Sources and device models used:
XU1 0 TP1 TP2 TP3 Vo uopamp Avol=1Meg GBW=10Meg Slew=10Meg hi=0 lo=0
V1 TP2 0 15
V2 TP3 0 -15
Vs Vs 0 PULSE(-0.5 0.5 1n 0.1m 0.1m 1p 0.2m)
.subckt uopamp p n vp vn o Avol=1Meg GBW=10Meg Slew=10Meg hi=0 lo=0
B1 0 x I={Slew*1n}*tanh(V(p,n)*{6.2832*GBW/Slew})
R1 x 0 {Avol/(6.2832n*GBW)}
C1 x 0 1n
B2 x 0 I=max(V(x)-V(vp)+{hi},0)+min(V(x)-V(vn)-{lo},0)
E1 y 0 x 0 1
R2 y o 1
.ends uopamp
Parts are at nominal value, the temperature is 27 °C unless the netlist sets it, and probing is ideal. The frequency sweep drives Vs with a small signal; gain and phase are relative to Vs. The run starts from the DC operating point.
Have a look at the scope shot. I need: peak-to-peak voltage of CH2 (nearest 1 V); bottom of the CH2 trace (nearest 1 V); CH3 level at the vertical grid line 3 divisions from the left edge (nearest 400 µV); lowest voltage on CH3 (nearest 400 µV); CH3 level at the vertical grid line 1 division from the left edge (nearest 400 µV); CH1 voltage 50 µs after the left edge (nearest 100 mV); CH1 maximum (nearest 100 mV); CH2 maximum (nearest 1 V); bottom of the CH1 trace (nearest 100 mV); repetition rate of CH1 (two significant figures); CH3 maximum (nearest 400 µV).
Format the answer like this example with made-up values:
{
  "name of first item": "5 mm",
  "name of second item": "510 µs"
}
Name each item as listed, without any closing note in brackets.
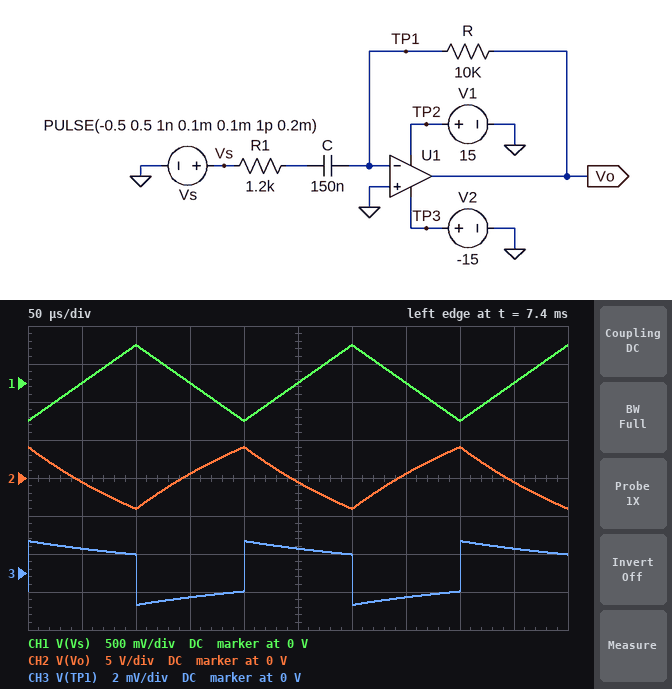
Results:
{
  "peak-to-peak voltage of CH2": "8 V",
  "bottom of the CH2 trace": "-4 V",
  "CH3 level at the vertical grid line 3 divisions from the left edge": "-1.2 mV",
  "lowest voltage on CH3": "-1.6 mV",
  "CH3 level at the vertical grid line 1 division from the left edge": "1.2 mV",
  "CH1 voltage 50 µs after the left edge": "0 V",
  "CH1 maximum": "500 mV",
  "CH2 maximum": "4 V",
  "bottom of the CH1 trace": "-500 mV",
  "repetition rate of CH1": "5.0 kHz",
  "CH3 maximum": "1.6 mV"
}
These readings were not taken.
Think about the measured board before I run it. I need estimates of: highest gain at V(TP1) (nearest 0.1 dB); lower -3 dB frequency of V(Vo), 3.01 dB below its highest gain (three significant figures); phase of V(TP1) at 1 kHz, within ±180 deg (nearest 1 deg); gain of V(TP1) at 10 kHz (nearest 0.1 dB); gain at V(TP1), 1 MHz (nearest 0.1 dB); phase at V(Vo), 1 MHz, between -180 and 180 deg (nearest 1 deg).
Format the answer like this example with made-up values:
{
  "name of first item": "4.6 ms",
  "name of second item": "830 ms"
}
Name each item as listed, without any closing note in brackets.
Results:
{
  "highest gain at V(TP1)": "-1.0 dB",
  "lower -3 dB frequency of V(Vo), 3.01 dB below its highest gain": "883 Hz",
  "phase of V(TP1) at 1 kHz, within ±180 deg": "131 deg",
  "gain of V(TP1) at 10 kHz": "-41.6 dB",
  "gain at V(TP1), 1 MHz": "-4.3 dB",
  "phase at V(Vo), 1 MHz, between -180 and 180 deg": "137 deg"
}
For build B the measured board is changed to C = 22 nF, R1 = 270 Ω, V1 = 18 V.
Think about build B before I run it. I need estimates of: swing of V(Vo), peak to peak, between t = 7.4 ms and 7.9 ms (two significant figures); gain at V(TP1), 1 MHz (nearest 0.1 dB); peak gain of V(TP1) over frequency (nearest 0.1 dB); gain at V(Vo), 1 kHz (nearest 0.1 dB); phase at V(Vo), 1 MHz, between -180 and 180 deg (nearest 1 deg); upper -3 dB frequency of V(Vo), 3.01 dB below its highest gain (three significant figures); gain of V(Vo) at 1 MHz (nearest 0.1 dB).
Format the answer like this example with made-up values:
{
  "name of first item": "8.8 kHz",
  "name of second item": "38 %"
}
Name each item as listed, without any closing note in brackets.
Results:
{
  "swing of V(Vo), peak to peak, between t = 7.4 ms and 7.9 ms": "4.4 V",
  "gain at V(TP1), 1 MHz": "-0.5 dB",
  "peak gain of V(TP1) over frequency": "-0.2 dB",
  "gain at V(Vo), 1 kHz": "2.8 dB",
  "phase at V(Vo), 1 MHz, between -180 and 180 deg": "105 deg",
  "upper -3 dB frequency of V(Vo), 3.01 dB below its highest gain": "288 kHz",
  "gain of V(Vo) at 1 MHz": "19.5 dB"
}
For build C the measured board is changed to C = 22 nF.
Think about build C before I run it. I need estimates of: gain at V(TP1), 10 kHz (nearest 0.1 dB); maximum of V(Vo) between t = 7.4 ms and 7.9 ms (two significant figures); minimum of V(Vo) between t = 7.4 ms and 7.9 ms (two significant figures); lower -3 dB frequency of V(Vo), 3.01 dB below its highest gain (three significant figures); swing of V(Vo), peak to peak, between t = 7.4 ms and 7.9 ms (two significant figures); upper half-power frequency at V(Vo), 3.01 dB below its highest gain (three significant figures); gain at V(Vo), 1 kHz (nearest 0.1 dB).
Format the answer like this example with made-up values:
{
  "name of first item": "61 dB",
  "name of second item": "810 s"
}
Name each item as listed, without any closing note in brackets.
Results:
{
  "gain at V(TP1), 10 kHz": "-42.9 dB",
  "maximum of V(Vo) between t = 7.4 ms and 7.9 ms": "2.1 V",
  "minimum of V(Vo) between t = 7.4 ms and 7.9 ms": "-2.1 V",
  "lower -3 dB frequency of V(Vo), 3.01 dB below its highest gain": "5.99 kHz",
  "swing of V(Vo), peak to peak, between t = 7.4 ms and 7.9 ms": "4.2 V",
  "upper half-power frequency at V(Vo), 3.01 dB below its highest gain": "1.08 MHz",
  "gain at V(Vo), 1 kHz": "2.7 dB"
}
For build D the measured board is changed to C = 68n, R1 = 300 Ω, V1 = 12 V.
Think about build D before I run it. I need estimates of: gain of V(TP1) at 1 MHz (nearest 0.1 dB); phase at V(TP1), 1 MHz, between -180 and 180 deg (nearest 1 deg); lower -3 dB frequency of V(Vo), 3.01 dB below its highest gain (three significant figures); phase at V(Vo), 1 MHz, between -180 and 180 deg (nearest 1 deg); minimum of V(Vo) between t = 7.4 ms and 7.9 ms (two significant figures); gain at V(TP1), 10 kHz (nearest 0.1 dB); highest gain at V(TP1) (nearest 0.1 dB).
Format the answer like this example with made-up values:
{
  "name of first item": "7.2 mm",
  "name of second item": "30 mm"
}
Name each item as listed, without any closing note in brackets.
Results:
{
  "gain of V(TP1) at 1 MHz": "-0.6 dB",
  "phase at V(TP1), 1 MHz, between -180 and 180 deg": "16 deg",
  "lower -3 dB frequency of V(Vo), 3.01 dB below its highest gain": "7.60 kHz",
  "phase at V(Vo), 1 MHz, between -180 and 180 deg": "106 deg",
  "minimum of V(Vo) between t = 7.4 ms and 7.9 ms": "-6.7 V",
  "gain at V(TP1), 10 kHz": "-31.5 dB",
  "highest gain at V(TP1)": "-0.3 dB"
}
